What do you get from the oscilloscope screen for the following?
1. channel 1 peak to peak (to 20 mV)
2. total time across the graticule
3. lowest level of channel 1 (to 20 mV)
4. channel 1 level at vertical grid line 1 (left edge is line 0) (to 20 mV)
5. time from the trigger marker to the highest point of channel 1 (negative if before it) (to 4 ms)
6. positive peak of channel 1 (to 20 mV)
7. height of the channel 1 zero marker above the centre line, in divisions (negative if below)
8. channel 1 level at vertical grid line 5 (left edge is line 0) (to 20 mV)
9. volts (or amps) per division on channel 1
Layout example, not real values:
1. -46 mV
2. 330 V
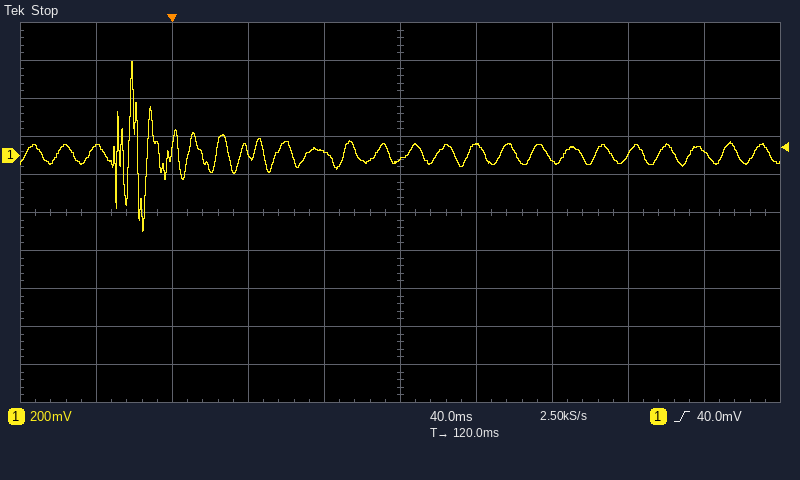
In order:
1. 900 mV
2. 400 ms
3. -400 mV
4. 40 mV
5. -20 ms
6. 500 mV
7. +1.5 div
8. -20 mV
9. 200 mV
